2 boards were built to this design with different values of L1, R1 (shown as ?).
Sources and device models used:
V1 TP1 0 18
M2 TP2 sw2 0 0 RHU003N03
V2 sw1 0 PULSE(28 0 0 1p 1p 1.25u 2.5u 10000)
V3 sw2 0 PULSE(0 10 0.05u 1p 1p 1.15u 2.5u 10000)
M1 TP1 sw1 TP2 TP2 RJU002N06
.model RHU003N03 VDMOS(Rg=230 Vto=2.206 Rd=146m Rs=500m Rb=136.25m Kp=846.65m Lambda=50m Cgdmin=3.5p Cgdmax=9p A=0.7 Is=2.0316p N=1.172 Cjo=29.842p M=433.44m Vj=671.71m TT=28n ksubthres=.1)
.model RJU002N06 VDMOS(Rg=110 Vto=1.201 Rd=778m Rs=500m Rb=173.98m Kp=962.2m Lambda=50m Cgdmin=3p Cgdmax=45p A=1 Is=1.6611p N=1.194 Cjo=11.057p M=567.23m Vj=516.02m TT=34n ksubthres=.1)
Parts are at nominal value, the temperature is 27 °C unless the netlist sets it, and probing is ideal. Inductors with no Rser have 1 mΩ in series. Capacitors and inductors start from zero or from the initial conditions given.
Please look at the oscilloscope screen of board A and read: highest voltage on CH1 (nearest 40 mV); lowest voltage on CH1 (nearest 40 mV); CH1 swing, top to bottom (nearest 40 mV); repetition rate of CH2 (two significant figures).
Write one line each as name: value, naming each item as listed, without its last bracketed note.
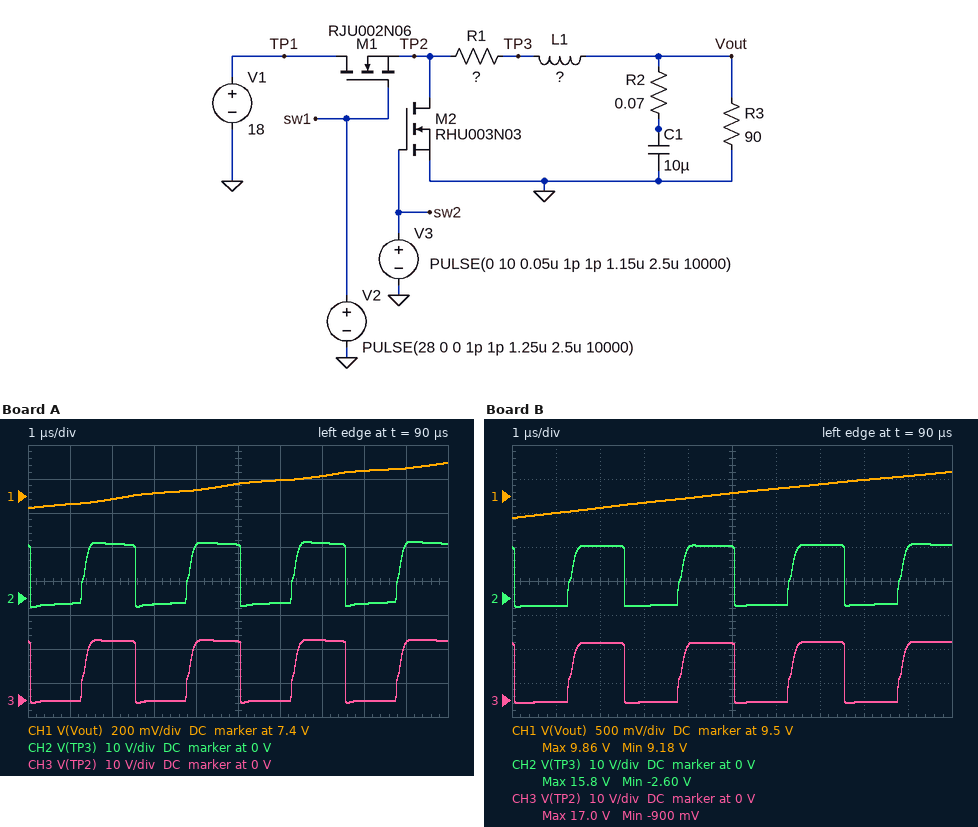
highest voltage on CH1: 7.60 V
lowest voltage on CH1: 7.32 V
CH1 swing, top to bottom: 280 mV
repetition rate of CH2: 400 kHz
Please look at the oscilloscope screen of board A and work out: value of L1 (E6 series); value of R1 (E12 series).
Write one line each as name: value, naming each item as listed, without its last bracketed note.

value of L1: 68 µH
value of R1: 3.9 Ω
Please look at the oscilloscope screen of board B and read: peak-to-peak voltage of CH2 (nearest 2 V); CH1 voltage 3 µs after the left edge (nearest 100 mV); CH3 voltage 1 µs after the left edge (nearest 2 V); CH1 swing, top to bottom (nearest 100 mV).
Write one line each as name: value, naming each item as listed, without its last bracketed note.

peak-to-peak voltage of CH2: 18 V
CH1 voltage 3 µs after the left edge: 9.4 V
CH3 voltage 1 µs after the left edge: 0 V
CH1 swing, top to bottom: 700 mV
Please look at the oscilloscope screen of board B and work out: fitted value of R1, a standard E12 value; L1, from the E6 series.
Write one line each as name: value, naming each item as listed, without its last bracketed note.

fitted value of R1, a standard E12 value: 1.8 Ω
L1, from the E6 series: 150 µH
